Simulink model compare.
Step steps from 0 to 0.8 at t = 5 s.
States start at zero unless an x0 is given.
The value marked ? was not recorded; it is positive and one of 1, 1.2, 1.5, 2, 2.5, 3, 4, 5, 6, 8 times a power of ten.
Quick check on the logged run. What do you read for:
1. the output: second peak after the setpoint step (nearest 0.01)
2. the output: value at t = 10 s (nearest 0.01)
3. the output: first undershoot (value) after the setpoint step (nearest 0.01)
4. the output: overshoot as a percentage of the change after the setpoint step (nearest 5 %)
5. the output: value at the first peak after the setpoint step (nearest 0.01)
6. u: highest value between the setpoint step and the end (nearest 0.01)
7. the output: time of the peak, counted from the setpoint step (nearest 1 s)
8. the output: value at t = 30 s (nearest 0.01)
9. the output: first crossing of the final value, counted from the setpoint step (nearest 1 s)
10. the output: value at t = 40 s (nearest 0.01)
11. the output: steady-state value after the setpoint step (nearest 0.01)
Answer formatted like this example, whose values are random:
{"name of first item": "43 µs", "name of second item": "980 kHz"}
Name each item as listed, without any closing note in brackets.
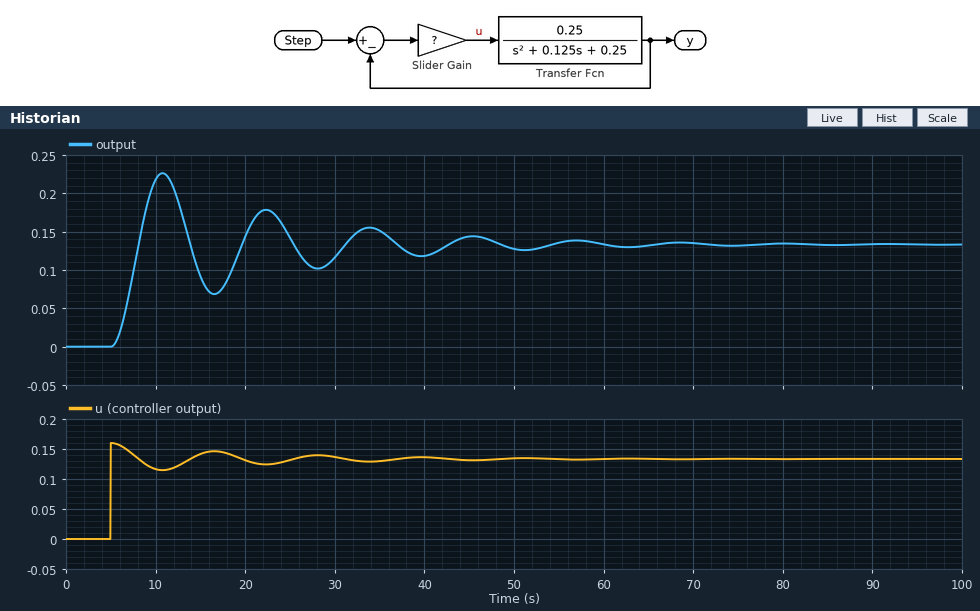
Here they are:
{"the output: second peak after the setpoint step": "0.18", "the output: value at t = 10 s": "0.22", "the output: first undershoot (value) after the setpoint step": "0.07", "the output: overshoot as a percentage of the change after the setpoint step": "70 %", "the output: value at the first peak after the setpoint step": "0.23", "u: highest value between the setpoint step and the end": "0.16", "the output: time of the peak, counted from the setpoint step": "6 s", "the output: value at t = 30 s": "0.12", "the output: first crossing of the final value, counted from the setpoint step": "3 s", "the output: value at t = 40 s": "0.12", "the output: steady-state value after the setpoint step": "0.13"}
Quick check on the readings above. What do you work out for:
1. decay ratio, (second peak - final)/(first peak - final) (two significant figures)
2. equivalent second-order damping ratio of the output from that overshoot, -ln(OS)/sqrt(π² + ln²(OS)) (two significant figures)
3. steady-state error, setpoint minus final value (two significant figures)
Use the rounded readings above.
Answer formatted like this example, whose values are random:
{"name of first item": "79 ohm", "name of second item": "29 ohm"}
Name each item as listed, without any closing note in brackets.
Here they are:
{"decay ratio, (second peak - final)/(first peak - final)": "0.50", "equivalent second-order damping ratio of the output from that overshoot, -ln(OS)/sqrt(π² + ln²(OS))": "0.11", "steady-state error, setpoint minus final value": "0.67"}
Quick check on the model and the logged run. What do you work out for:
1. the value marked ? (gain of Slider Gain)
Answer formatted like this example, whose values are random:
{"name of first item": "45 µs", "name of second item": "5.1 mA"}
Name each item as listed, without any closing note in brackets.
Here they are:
{"the value marked ?": "0.2"}
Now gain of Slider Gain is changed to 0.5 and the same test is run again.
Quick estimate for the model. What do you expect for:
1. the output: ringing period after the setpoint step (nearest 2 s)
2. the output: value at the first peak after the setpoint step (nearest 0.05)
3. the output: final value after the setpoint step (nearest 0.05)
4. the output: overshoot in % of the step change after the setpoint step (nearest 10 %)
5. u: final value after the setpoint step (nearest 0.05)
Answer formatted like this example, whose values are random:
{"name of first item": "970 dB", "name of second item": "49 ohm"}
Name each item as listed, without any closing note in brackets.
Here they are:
{"the output: ringing period after the setpoint step": "10 s", "the output: value at the first peak after the setpoint step": "0.45", "the output: final value after the setpoint step": "0.25", "the output: overshoot in % of the step change after the setpoint step": "70 %", "u: final value after the setpoint step": "0.25"}
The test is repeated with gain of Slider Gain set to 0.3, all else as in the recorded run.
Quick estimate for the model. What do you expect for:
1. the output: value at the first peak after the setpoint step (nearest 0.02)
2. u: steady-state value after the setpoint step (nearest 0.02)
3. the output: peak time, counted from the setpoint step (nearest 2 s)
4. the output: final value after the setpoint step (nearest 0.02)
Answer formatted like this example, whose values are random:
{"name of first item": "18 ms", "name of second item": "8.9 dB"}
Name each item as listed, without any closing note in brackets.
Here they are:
{"the output: value at the first peak after the setpoint step": "0.32", "u: steady-state value after the setpoint step": "0.18", "the output: peak time, counted from the setpoint step": "6 s", "the output: final value after the setpoint step": "0.18"}
